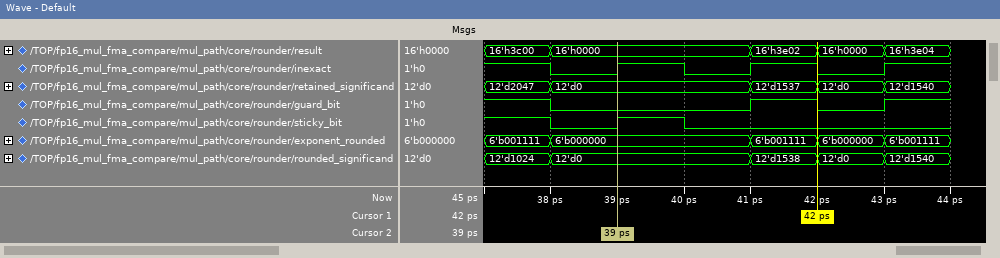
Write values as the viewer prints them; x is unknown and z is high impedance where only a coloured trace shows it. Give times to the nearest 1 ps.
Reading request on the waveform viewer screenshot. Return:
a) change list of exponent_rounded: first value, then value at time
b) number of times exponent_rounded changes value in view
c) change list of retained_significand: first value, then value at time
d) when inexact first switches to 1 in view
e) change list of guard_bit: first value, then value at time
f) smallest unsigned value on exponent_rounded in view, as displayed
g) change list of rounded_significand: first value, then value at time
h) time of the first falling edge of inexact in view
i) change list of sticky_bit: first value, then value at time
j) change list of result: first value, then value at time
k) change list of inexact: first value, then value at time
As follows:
6'b001111, 6'b000000 at 38 ps, 6'b001111 at 41 ps, 6'b000000 at 42 ps, 6'b001111 at 43 ps
4
12'd2047, 12'd0 at 38 ps, 12'd1537 at 41 ps, 12'd0 at 42 ps, 12'd1540 at 43 ps
39 ps
1, 0 at 38 ps, 1 at 41 ps, 0 at 42 ps, 1 at 43 ps
6'b000000
12'd1024, 12'd0 at 38 ps, 12'd1538 at 41 ps, 12'd0 at 42 ps, 12'd1540 at 43 ps
38 ps
1, 0 at 38 ps, 1 at 39 ps, 0 at 40 ps
16'h3c00, 16'h0000 at 38 ps, 16'h3e02 at 41 ps, 16'h0000 at 42 ps, 16'h3e04 at 43 ps
1, 0 at 38 ps, 1 at 39 ps, 0 at 40 ps, 1 at 41 ps, 0 at 42 ps, 1 at 43 ps
